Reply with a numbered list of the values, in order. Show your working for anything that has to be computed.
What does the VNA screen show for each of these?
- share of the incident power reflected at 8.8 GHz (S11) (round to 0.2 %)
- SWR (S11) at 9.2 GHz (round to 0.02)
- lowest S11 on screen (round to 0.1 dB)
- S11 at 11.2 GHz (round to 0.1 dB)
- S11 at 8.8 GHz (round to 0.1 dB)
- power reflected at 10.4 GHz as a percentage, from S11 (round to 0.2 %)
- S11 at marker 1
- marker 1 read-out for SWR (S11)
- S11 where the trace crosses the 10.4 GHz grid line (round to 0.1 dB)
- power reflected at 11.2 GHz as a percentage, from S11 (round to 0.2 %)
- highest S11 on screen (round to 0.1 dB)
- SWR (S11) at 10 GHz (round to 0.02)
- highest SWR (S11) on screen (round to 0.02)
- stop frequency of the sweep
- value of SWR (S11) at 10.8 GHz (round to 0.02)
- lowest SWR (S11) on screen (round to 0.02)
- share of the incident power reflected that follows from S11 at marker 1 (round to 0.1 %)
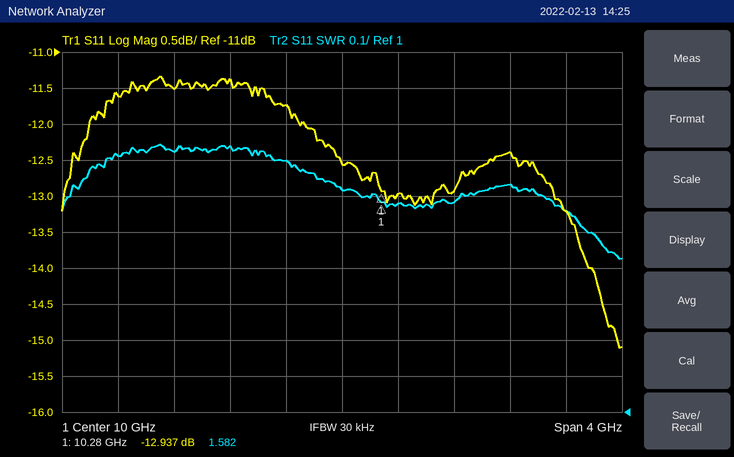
1. 10^(-11.5/10) ≈ 7.08 %, so 7.0 % to the nearest 0.2 %
2. 1.74
3. -15.1 dB
4. -12.4 dB
5. -11.5 dB
6. 10^(-13/10) ≈ 5.0 %
7. -12.937 dB
8. 1.582
9. -13.0 dB
10. 10^(-12.4/10) ≈ 5.8 %
11. -11.3 dB
12. 1.62
13. 1.74
14. 12 GHz
15. 1.58
16. 1.42
17. 10^(-12.937/10) ≈ 5.1 %
